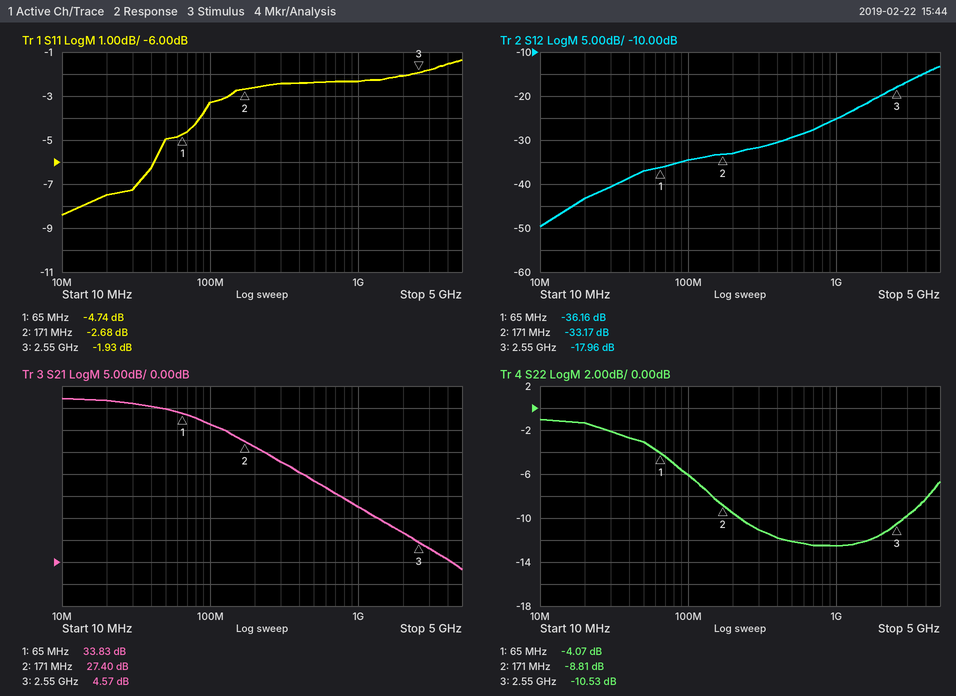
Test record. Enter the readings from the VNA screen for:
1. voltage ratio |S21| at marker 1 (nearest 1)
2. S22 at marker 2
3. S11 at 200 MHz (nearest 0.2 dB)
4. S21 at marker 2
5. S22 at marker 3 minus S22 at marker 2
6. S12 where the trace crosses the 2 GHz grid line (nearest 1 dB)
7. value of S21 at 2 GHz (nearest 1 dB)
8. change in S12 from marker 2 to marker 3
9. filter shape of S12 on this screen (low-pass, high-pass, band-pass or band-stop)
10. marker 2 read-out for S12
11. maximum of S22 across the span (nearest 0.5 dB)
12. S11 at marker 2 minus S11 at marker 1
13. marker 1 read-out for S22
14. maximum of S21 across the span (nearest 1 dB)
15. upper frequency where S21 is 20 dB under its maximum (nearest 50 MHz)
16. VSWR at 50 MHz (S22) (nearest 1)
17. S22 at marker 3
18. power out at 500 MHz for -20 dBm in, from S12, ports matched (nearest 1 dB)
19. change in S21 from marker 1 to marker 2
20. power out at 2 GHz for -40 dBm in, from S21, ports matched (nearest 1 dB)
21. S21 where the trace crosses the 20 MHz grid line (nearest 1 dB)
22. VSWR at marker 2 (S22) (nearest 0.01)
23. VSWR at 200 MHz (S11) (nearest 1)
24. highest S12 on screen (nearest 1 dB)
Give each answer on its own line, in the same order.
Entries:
49
-8.81 dB
-2.6 dB
27.40 dB
-1.72 dB
-20 dB
7 dB
15.21 dB
high-pass
-33.17 dB
-1.0 dB
2.06 dB
-4.07 dB
37 dB
600 MHz
6
-10.53 dB
-49 dBm
-6.43 dB
-33 dBm
37 dB
2.14
7
-13 dB
